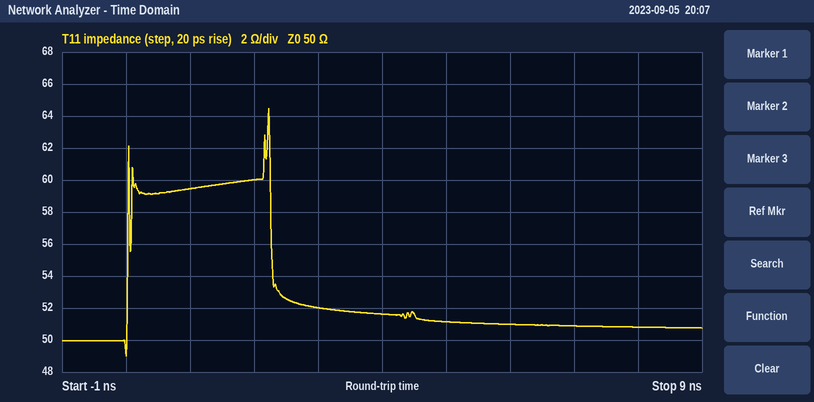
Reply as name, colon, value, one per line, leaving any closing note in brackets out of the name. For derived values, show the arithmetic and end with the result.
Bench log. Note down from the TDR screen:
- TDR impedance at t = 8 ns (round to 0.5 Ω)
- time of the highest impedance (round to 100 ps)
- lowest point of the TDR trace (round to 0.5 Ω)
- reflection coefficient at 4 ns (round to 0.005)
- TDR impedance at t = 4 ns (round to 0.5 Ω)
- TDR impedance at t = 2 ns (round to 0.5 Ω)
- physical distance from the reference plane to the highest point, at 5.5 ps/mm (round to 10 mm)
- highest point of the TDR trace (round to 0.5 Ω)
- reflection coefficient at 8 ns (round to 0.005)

TDR impedance at t = 8 ns: 51.0 Ω
time of the highest impedance: 2.2 ns
lowest point of the TDR trace: 49.0 Ω
reflection coefficient at 4 ns: (51.5 − 50)/(51.5 + 50) ≈ +0.015
TDR impedance at t = 4 ns: 51.5 Ω
TDR impedance at t = 2 ns: 60.0 Ω
physical distance from the reference plane to the highest point, at 5.5 ps/mm: 2.2 ns / 2 / 5.5 ps/mm ≈ 200 mm
highest point of the TDR trace: 64.5 Ω
reflection coefficient at 8 ns: (51 − 50)/(51 + 50) ≈ +0.010
